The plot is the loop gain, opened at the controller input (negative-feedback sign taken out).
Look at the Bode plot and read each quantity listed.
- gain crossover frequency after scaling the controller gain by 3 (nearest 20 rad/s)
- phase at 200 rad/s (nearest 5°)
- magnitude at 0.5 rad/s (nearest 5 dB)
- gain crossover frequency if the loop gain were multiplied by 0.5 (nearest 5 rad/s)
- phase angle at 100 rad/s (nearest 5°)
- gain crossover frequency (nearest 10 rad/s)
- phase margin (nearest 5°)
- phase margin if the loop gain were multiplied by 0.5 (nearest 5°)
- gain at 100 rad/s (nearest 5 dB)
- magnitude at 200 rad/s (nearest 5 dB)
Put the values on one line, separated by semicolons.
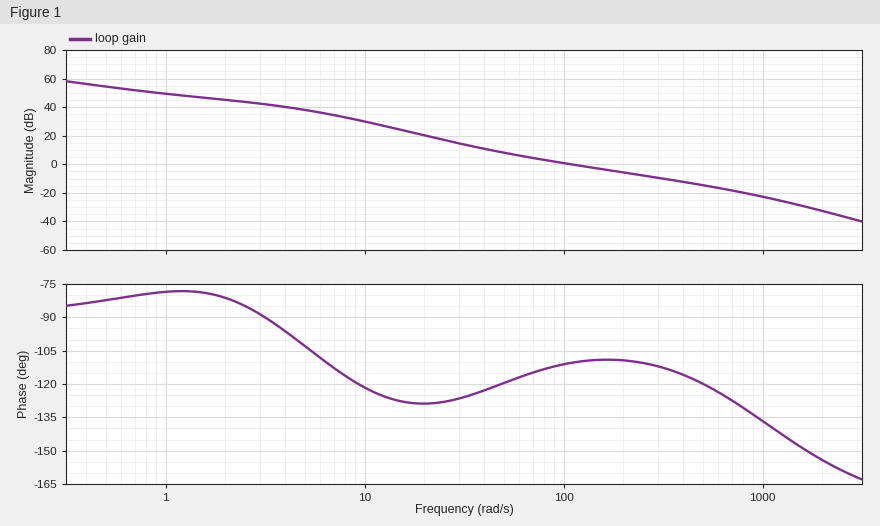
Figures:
300 rad/s; -110°; 55 dB; 60 rad/s; -110°; 110 rad/s; 70°; 65°; 0 dB; -5 dB
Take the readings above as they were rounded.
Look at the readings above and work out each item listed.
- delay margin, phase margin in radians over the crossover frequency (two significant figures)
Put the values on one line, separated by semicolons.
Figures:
0.011 s
